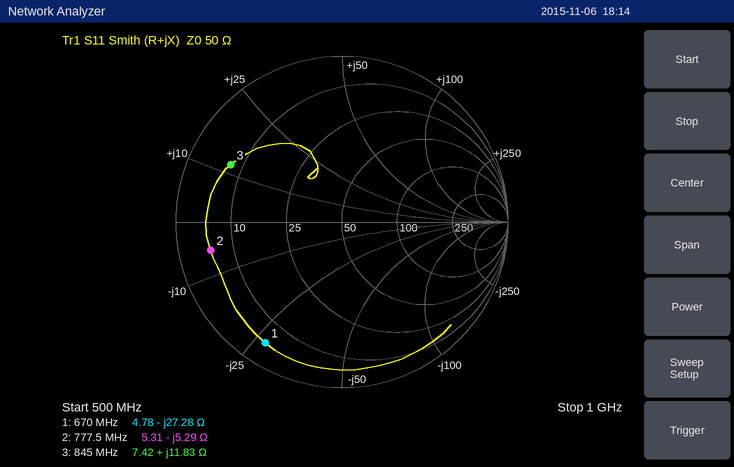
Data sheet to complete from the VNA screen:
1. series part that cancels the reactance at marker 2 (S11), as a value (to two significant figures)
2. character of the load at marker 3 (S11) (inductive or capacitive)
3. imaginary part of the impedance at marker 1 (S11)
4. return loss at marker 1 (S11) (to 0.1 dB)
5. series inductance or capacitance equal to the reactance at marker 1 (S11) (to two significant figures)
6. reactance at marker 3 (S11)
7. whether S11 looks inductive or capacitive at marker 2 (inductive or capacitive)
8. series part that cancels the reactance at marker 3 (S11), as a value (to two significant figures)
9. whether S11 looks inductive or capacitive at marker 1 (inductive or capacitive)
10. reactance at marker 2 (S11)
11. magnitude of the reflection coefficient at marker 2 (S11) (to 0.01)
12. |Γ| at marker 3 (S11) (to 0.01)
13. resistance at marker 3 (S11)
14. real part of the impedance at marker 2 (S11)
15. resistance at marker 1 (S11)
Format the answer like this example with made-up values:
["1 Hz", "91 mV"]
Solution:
["1.1 nH", "inductive", "-27.28 Ω", "1.3 dB", "8.7 pF", "+11.83 Ω", "capacitive", "16 pF", "capacitive", "-5.29 Ω", "0.81", "0.75", "7.42 Ω", "5.31 Ω", "4.78 Ω"]
